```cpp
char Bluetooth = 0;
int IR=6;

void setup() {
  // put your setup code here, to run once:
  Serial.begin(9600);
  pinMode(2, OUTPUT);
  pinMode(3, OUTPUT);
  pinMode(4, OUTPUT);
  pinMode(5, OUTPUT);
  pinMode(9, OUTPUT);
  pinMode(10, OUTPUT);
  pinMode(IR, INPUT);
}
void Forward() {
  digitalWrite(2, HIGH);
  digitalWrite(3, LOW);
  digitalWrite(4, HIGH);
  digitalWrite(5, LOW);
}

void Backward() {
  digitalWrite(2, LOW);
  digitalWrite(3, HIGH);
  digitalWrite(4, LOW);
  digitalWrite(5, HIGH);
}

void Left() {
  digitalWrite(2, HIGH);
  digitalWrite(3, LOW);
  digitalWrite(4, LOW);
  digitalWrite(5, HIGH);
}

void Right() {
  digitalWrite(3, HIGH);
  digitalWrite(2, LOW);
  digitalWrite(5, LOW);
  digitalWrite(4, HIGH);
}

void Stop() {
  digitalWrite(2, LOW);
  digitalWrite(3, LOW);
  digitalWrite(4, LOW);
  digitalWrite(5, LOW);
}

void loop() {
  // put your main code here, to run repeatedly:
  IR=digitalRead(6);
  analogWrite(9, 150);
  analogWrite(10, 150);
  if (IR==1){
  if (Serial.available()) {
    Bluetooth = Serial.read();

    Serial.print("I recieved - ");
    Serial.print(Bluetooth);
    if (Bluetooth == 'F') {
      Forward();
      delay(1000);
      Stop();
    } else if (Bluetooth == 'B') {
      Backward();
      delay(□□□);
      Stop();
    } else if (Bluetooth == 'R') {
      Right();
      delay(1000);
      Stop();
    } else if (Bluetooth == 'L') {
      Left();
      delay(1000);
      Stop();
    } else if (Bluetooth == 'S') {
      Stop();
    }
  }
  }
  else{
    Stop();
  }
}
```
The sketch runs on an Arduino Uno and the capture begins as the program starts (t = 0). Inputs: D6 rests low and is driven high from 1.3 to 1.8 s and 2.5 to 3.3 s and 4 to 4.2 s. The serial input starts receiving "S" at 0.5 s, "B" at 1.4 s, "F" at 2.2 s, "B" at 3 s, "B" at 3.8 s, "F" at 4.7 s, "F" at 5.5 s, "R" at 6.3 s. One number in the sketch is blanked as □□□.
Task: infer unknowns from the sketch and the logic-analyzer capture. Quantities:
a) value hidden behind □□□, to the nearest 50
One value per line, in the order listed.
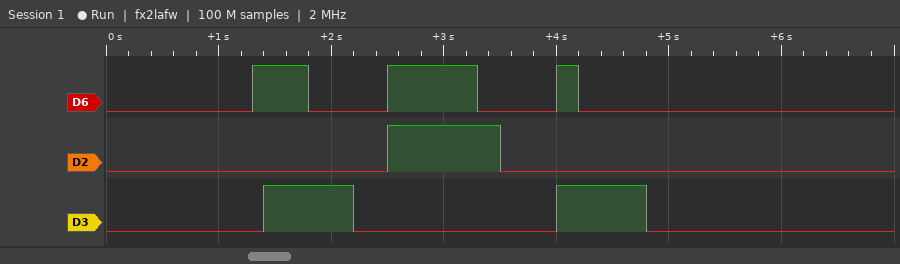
800
